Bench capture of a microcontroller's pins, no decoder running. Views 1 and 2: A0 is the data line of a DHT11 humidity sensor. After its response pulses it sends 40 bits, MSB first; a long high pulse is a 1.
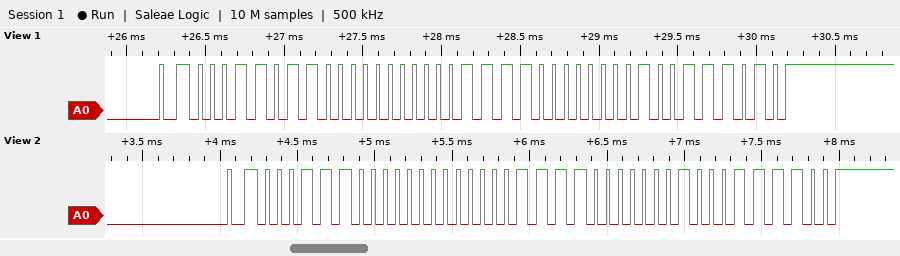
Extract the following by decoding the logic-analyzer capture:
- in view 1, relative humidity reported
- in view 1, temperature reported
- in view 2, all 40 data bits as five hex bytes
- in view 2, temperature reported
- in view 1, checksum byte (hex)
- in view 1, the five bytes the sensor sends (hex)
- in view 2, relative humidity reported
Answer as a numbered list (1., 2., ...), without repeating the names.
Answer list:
1. 27 %
2. 30.1 °C
3. 1C 00 1E 02 3C
4. 30.2 °C
5. 0x3A
6. 1B 00 1E 01 3A
7. 28 %
